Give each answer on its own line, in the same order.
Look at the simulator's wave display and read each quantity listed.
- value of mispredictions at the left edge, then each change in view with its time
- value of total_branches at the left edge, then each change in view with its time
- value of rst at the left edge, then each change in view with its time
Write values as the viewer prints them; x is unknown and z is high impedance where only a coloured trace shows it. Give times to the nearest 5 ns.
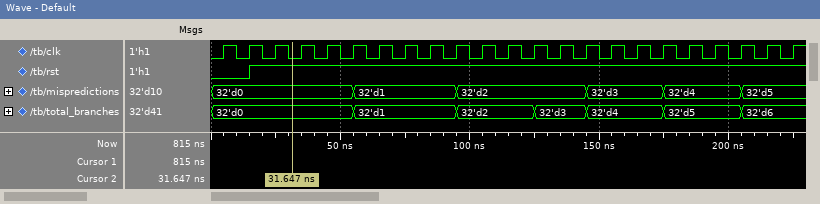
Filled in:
32'd0, 32'd1 at 55 ns, 32'd2 at 95 ns, 32'd3 at 145 ns, 32'd4 at 175 ns, 32'd5 at 205 ns
32'd0, 32'd1 at 55 ns, 32'd2 at 95 ns, 32'd3 at 125 ns, 32'd4 at 145 ns, 32'd5 at 175 ns, 32'd6 at 205 ns
0, 1 at 15 ns
